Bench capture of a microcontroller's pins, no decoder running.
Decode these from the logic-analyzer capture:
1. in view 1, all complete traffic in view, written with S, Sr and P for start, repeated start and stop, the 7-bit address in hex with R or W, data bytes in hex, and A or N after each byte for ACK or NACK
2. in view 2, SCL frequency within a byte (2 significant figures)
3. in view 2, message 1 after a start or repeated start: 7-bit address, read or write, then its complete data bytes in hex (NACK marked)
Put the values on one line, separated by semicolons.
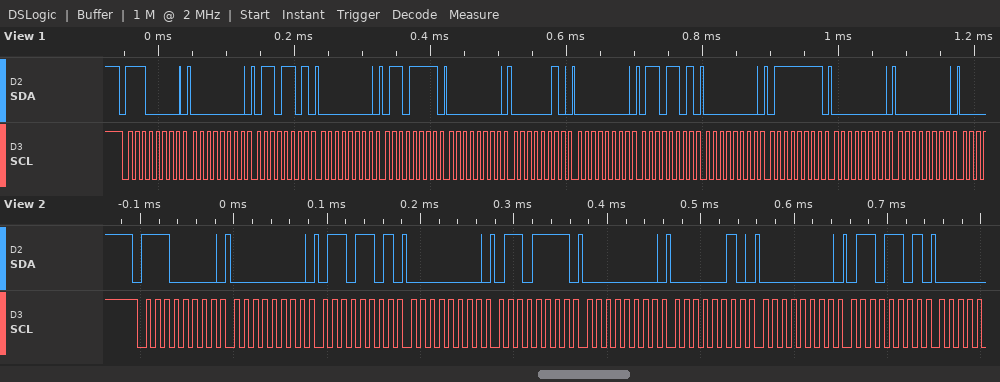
S 70W A 00 A 6D A 00 A 6F A 00 A 02 A 00 A 6D A 00 A 7F A 00 A 00 A; 100 kHz; 0x70 write: 00 6D 00 6F 00 02 00 6D
